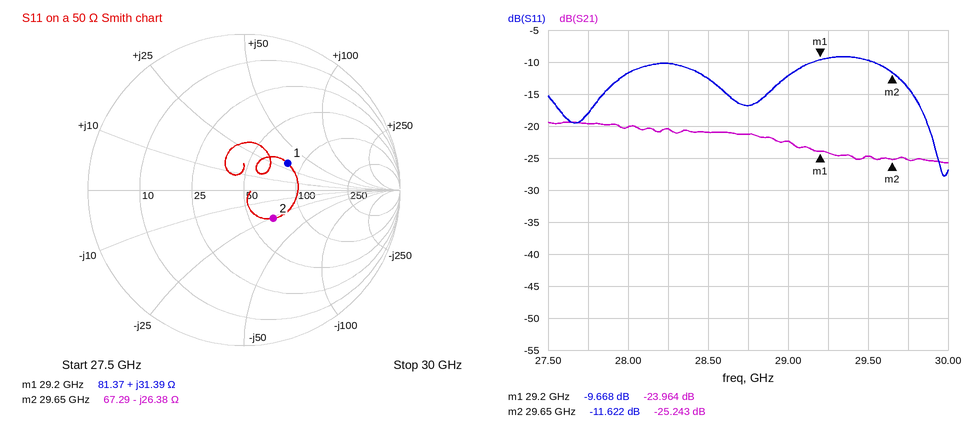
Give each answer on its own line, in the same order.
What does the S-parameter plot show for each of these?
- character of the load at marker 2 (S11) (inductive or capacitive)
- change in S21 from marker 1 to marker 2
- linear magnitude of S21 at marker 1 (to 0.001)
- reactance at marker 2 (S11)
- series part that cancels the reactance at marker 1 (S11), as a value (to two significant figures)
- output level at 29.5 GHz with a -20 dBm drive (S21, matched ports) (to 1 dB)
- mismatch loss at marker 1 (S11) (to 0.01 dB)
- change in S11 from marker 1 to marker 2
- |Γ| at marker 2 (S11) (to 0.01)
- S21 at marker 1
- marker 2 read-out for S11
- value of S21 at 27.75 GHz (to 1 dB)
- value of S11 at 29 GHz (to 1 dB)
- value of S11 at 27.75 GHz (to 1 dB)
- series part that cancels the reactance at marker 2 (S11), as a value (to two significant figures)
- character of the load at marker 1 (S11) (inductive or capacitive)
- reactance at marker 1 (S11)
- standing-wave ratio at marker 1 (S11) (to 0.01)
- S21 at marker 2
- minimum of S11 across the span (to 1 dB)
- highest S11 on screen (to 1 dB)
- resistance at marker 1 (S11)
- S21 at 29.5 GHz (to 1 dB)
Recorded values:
capacitive
-1.279 dB
0.063
-26.38 Ω
170 fF
-45 dBm
0.50 dB
-1.954 dB
0.26
-23.964 dB
-11.622 dB
-20 dB
-12 dB
-18 dB
140 pH
inductive
+31.39 Ω
1.98
-25.243 dB
-28 dB
-9 dB
81.37 Ω
-25 dB
